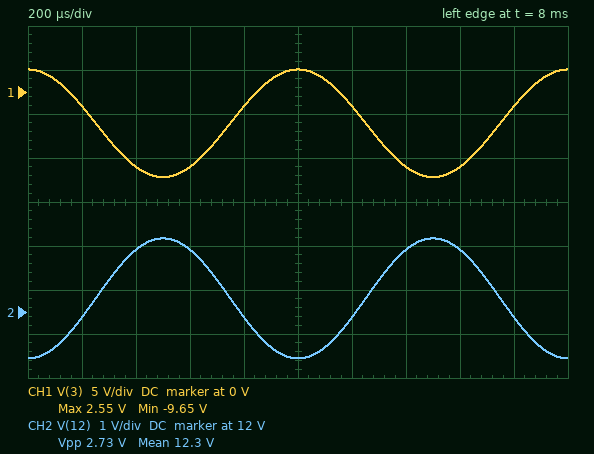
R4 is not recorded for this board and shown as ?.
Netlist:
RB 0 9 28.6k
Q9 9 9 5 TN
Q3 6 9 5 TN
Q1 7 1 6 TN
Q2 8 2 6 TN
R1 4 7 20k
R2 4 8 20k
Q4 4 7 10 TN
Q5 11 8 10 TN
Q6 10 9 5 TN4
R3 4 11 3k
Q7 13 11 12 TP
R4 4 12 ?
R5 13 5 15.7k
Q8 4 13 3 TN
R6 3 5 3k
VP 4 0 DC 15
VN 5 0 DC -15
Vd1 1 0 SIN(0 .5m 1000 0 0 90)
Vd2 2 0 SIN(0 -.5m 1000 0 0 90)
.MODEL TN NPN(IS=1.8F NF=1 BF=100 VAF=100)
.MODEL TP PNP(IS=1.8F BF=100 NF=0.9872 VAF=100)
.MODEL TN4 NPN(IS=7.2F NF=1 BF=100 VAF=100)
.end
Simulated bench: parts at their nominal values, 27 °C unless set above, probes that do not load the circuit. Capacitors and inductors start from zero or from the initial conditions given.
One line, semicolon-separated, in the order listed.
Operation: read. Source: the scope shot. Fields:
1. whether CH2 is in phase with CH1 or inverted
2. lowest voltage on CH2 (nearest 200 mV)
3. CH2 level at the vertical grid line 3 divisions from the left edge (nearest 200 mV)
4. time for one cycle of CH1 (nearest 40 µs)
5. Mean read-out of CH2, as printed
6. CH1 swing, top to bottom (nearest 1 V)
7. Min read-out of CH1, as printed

inverted; 11.0 V; 13.4 V; 1.00 ms; 12.3 V; 12 V; -9.65 V
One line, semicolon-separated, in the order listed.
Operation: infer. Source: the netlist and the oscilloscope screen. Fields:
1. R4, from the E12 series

3.3 kΩ
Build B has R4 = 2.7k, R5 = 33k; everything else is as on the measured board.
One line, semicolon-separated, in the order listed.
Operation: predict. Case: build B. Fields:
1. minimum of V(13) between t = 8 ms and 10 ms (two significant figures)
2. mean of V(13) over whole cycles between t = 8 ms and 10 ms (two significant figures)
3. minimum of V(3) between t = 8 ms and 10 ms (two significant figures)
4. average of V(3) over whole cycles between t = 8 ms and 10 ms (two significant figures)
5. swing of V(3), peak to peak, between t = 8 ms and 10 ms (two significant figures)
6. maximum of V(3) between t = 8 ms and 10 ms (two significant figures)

-360 mV; 8.4 V; -1.1 V; 7.7 V; 13 V; 12 V
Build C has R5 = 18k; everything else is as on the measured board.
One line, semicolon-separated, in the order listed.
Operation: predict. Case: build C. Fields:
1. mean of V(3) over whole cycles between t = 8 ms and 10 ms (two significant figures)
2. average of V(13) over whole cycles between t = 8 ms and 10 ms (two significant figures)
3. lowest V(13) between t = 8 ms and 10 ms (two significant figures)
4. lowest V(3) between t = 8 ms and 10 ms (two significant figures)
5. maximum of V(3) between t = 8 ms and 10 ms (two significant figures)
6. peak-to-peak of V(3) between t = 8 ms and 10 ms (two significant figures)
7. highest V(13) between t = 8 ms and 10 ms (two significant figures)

-1.9 V; -1.1 V; -8.1 V; -8.8 V; 5.1 V; 14 V; 5.8 V
